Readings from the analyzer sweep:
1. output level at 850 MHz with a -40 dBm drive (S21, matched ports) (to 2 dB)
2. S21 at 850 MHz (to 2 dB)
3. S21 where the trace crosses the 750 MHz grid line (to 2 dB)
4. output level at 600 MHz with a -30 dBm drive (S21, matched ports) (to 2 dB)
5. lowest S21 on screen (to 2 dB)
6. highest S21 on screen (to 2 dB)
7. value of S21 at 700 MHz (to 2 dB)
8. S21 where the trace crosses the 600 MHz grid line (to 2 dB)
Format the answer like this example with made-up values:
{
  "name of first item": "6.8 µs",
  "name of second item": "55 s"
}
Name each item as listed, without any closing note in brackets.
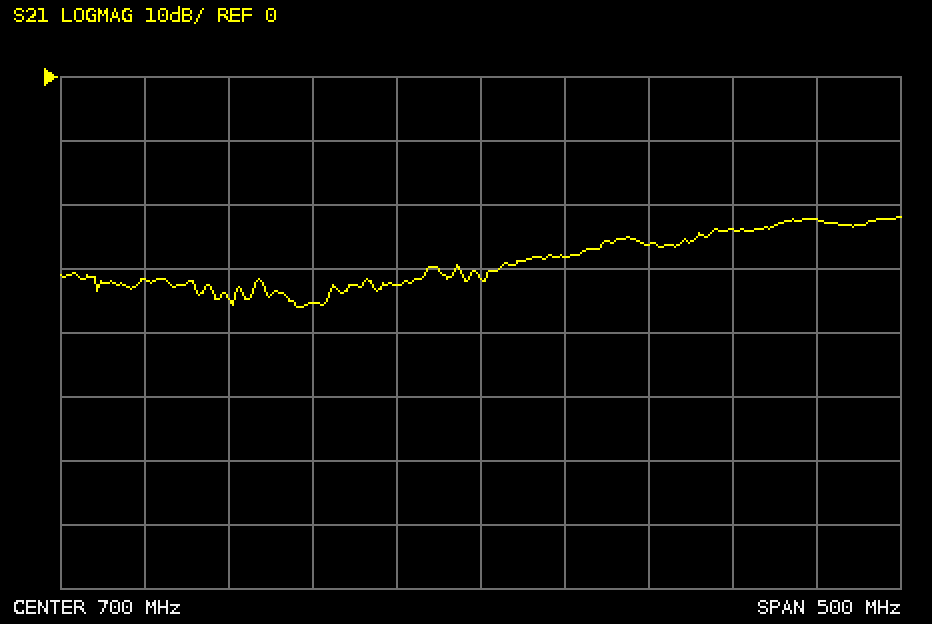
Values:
{
  "output level at 850 MHz with a -40 dBm drive (S21, matched ports)": "-64 dBm",
  "S21 at 850 MHz": "-24 dB",
  "S21 where the trace crosses the 750 MHz grid line": "-28 dB",
  "output level at 600 MHz with a -30 dBm drive (S21, matched ports)": "-66 dBm",
  "lowest S21 on screen": "-36 dB",
  "highest S21 on screen": "-22 dB",
  "value of S21 at 700 MHz": "-32 dB",
  "S21 where the trace crosses the 600 MHz grid line": "-36 dB"
}
